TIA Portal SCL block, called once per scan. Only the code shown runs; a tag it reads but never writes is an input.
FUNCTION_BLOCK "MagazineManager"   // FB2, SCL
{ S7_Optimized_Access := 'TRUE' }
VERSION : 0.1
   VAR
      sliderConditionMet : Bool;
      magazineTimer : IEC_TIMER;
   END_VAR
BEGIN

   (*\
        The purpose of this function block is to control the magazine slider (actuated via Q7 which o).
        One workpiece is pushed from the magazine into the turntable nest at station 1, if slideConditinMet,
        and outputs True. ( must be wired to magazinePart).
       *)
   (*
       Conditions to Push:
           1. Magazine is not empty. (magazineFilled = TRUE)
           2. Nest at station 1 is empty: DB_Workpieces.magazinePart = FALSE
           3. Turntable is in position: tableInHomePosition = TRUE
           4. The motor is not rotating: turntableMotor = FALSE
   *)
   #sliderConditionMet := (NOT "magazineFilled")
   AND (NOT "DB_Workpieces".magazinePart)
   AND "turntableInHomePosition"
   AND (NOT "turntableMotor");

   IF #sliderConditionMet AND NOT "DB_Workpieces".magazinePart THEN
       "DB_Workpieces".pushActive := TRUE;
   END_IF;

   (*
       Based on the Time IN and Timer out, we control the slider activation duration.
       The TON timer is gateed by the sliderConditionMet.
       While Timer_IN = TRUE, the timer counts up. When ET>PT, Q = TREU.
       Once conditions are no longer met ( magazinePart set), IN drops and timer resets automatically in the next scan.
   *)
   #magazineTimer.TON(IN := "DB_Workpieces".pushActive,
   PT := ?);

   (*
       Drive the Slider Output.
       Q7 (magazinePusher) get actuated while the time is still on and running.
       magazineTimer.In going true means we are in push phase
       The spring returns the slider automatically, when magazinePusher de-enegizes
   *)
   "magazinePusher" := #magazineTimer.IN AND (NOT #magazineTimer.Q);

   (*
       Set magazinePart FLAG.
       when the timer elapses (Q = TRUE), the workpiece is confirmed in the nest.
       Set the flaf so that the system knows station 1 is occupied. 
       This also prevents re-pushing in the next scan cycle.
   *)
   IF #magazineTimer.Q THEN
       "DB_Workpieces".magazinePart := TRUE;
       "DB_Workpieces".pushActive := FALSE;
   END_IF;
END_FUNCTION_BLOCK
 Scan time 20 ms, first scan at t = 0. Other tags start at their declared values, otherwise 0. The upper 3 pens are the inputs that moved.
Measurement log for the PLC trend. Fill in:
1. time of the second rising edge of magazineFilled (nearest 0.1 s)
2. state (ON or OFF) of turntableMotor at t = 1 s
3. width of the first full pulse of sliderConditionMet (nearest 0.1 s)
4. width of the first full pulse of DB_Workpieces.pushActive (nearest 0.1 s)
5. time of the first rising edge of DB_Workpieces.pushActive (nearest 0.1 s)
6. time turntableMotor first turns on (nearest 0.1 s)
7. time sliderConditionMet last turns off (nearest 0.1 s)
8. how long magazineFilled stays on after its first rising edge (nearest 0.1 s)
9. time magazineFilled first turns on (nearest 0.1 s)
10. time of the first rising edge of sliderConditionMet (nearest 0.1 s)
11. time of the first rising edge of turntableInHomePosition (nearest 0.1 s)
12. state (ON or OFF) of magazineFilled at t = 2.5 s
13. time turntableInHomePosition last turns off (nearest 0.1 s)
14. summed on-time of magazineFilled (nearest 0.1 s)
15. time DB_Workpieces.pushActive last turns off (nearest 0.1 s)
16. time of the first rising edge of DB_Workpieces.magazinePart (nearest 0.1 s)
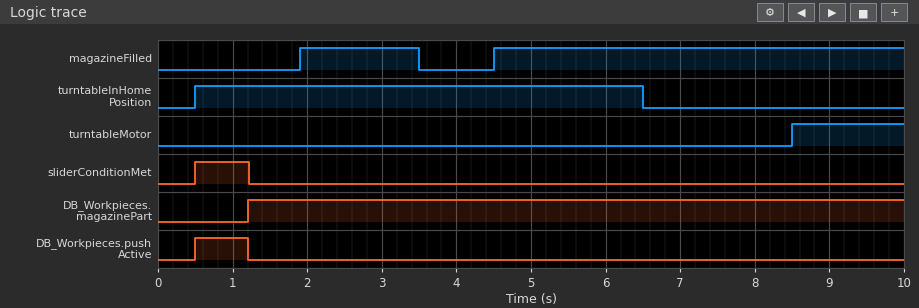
4.5 s
OFF
0.7 s
0.7 s
0.5 s
8.5 s
1.2 s
1.6 s
1.9 s
0.5 s
0.5 s
ON
6.5 s
7.1 s
1.2 s
1.2 s
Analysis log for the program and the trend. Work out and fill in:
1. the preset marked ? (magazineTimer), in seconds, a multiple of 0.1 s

0.7 s
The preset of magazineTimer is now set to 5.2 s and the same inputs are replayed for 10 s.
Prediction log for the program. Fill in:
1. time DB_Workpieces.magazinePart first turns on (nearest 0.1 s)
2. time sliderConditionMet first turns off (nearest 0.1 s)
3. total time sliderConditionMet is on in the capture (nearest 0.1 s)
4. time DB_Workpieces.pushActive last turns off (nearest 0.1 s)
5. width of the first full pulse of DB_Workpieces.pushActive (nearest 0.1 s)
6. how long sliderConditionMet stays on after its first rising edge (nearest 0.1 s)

5.7 s
1.9 s
2.4 s
5.7 s
5.2 s
1.4 s
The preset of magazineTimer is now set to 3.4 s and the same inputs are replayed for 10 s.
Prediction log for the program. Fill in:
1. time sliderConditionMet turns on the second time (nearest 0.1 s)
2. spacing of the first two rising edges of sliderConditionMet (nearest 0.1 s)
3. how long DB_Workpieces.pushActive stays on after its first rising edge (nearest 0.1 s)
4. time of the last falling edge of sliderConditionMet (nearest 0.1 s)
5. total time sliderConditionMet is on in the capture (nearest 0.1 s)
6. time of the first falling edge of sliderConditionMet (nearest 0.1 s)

3.5 s
3.0 s
3.4 s
3.9 s
1.8 s
1.9 s
